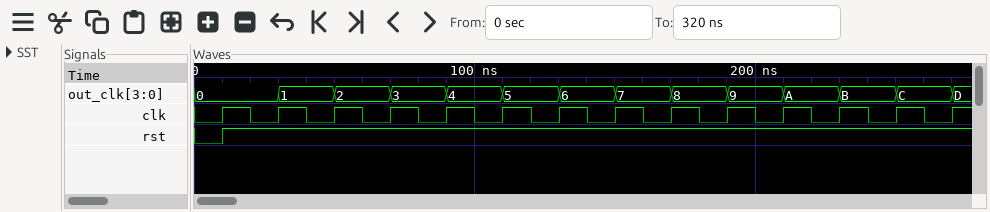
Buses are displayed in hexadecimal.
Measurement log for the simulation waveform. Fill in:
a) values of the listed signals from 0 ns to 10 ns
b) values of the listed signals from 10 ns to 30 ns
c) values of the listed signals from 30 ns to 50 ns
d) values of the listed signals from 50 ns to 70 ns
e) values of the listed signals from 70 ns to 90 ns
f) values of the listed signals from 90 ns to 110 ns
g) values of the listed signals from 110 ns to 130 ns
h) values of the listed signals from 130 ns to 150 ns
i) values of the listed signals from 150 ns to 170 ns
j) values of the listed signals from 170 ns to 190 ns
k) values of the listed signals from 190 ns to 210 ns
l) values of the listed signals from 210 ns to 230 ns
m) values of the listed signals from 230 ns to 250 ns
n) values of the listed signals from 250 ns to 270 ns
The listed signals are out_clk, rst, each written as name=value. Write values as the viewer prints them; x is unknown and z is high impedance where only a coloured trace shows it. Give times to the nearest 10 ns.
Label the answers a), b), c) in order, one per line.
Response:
a) out_clk=0, rst=0
b) out_clk=0, rst=1
c) out_clk=1, rst=1
d) out_clk=2, rst=1
e) out_clk=3, rst=1
f) out_clk=4, rst=1
g) out_clk=5, rst=1
h) out_clk=6, rst=1
i) out_clk=7, rst=1
j) out_clk=8, rst=1
k) out_clk=9, rst=1
l) out_clk=A, rst=1
m) out_clk=B, rst=1
n) out_clk=C, rst=1
